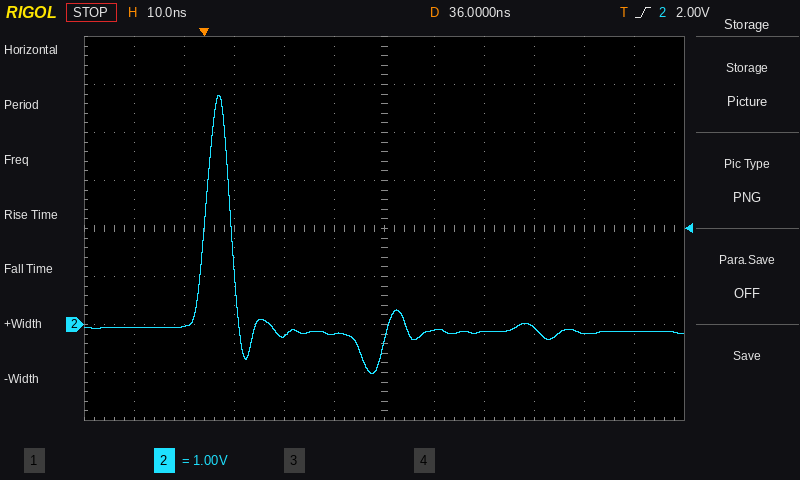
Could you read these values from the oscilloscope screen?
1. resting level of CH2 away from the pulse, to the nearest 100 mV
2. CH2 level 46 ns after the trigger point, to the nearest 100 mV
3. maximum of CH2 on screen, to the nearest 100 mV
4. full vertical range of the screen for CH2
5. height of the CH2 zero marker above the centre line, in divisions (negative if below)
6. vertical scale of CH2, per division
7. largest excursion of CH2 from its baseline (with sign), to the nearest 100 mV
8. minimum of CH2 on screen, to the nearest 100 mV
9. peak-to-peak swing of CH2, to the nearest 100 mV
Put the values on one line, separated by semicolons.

-100 mV; -100 mV; 4.8 V; 8 V; -2.0 div; 1 V; +4.9 V; -1.0 V; 5.8 V
